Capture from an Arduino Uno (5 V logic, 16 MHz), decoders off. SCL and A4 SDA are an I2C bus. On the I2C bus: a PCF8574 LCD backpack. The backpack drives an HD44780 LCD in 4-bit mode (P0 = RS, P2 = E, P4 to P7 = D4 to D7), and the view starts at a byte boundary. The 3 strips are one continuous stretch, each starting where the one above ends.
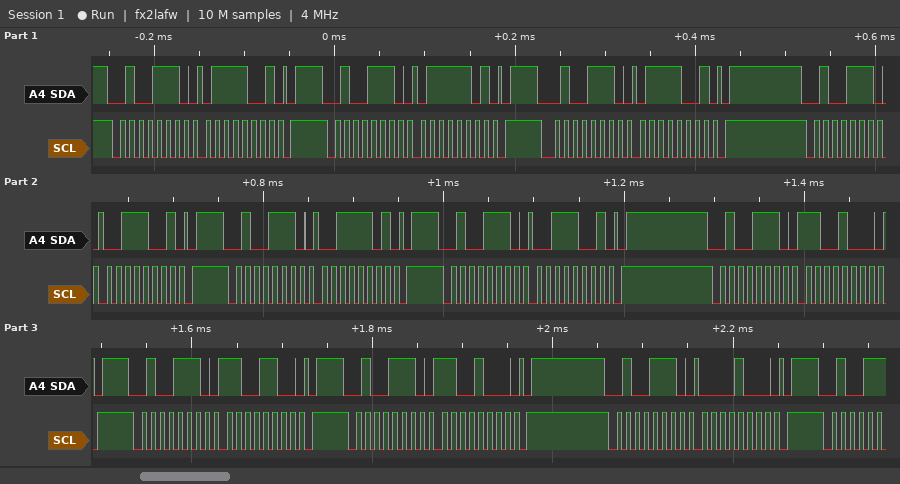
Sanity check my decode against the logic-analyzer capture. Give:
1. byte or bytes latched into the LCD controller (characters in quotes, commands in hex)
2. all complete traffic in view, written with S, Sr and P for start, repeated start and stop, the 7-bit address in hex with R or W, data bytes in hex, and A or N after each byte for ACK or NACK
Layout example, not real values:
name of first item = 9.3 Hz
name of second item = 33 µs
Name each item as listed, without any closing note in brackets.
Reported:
byte or bytes latched into the LCD controller = 's'
all complete traffic in view, written with S, Sr and P for start, repeated start and stop, the 7-bit address in hex with R or W, data bytes in hex, and A or N after each byte for ACK or NACK = S 27W A 79 A P S 27W A 7D A P S 27W A 79 A P S 27W A 39 A P S 27W A 3D A P S 27W A 39 A P S 27W A C8 A P S 27W A CC A P S 27W A C8 A P S 27W A 08 A P
